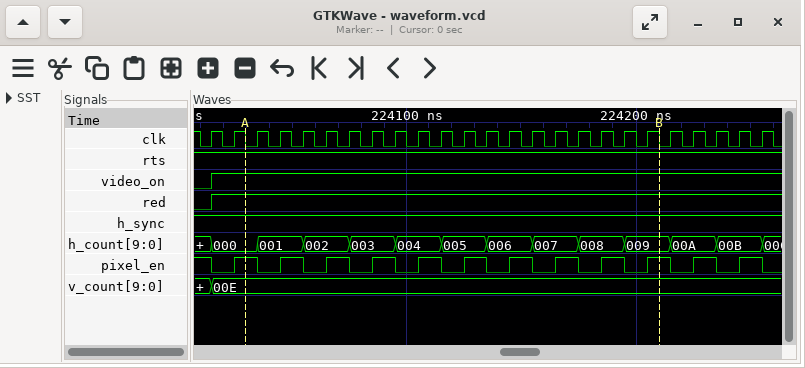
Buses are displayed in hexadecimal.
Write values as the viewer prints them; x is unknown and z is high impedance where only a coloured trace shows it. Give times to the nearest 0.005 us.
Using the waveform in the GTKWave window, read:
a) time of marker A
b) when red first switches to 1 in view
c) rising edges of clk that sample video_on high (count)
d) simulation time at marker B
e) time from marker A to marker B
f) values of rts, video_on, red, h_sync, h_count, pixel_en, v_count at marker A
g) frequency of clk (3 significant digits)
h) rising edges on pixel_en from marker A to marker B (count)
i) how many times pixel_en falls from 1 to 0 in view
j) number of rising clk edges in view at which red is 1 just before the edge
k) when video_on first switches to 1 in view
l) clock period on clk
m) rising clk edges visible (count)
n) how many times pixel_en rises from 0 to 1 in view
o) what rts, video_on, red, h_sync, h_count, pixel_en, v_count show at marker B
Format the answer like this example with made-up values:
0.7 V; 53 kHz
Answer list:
224.03 us; 224.015 us; 24; 224.21 us; 0.18 us; rts=1, video_on=1, red=1, h_sync=1, h_count=000, pixel_en=1, v_count=00E; 100 MHz; 9; 13; 24; 224.015 us; 0.01 us; 25; 12; rts=1, video_on=1, red=1, h_sync=1, h_count=009, pixel_en=1, v_count=00E
